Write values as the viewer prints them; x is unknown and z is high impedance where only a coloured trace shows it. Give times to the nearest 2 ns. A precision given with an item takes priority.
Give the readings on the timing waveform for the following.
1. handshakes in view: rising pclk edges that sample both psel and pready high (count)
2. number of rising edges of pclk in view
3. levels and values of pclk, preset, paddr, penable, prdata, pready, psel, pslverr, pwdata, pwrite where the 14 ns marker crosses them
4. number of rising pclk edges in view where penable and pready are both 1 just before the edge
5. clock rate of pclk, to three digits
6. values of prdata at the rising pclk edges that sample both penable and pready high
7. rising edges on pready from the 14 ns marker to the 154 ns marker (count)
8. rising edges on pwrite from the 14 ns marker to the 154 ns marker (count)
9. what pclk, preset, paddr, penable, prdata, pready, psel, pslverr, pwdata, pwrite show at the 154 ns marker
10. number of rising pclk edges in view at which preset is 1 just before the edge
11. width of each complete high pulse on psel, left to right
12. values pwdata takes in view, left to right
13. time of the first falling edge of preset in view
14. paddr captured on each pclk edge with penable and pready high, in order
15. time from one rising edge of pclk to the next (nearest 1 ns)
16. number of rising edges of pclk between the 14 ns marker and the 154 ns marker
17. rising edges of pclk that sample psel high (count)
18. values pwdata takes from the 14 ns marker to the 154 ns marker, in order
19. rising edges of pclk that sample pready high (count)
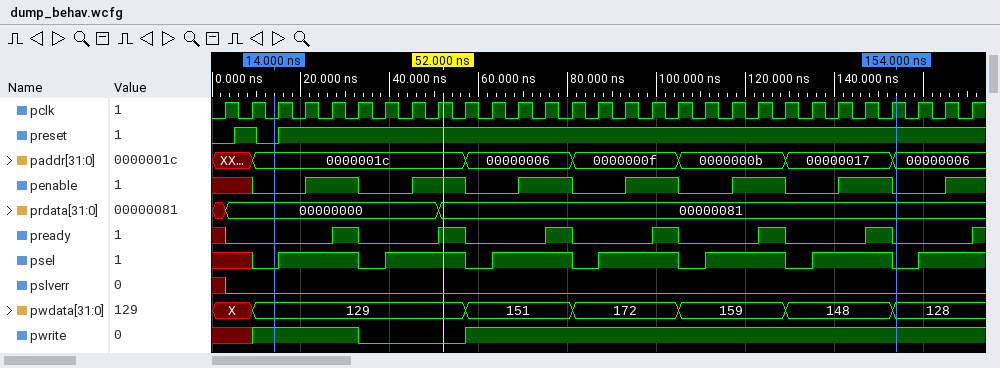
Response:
6
29
pclk=0, preset=0, paddr=0000001c, penable=0, prdata=00000000, pready=0, psel=0, pslverr=0, pwdata=129, pwrite=1
6
167 MHz
00000000, 00000081, 00000081, 00000081, 00000081, 00000081
6
1
pclk=1, preset=1, paddr=00000006, penable=0, prdata=00000081, pready=0, psel=0, pslverr=0, pwdata=128, pwrite=1
27
18 ns, 18 ns, 18 ns, 18 ns, 18 ns, 18 ns
X, 129, 151, 172, 159, 148, 128
10 ns
0000001c, 0000001c, 00000006, 0000000f, 0000000b, 00000017
6 ns
24
20
129, 151, 172, 159, 148, 128
6
